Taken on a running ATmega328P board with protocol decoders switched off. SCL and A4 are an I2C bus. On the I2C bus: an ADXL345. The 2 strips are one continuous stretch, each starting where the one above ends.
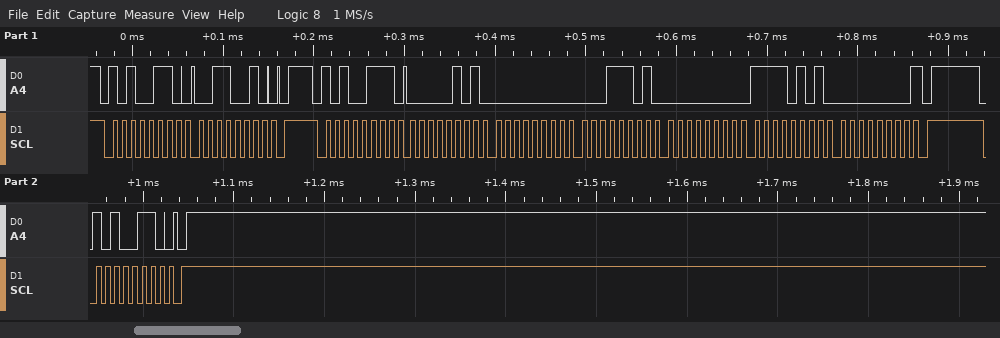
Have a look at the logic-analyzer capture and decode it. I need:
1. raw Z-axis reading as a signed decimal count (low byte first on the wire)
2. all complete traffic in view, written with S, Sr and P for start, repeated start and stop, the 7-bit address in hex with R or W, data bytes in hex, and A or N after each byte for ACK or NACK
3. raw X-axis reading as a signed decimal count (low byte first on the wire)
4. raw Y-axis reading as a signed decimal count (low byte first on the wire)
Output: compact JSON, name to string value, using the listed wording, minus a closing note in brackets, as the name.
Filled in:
{"raw Z-axis reading as a signed decimal count": "245", "all complete traffic in view, written with S, Sr and P for start, repeated start and stop, the 7-bit address in hex with R or W, data bytes in hex, and A or N after each byte for ACK or NACK": "S 53W A 32 A P S 53R A 05 A 00 A 1D A 00 A F5 A 00 N P S 53W A P", "raw X-axis reading as a signed decimal count": "5", "raw Y-axis reading as a signed decimal count": "29"}
